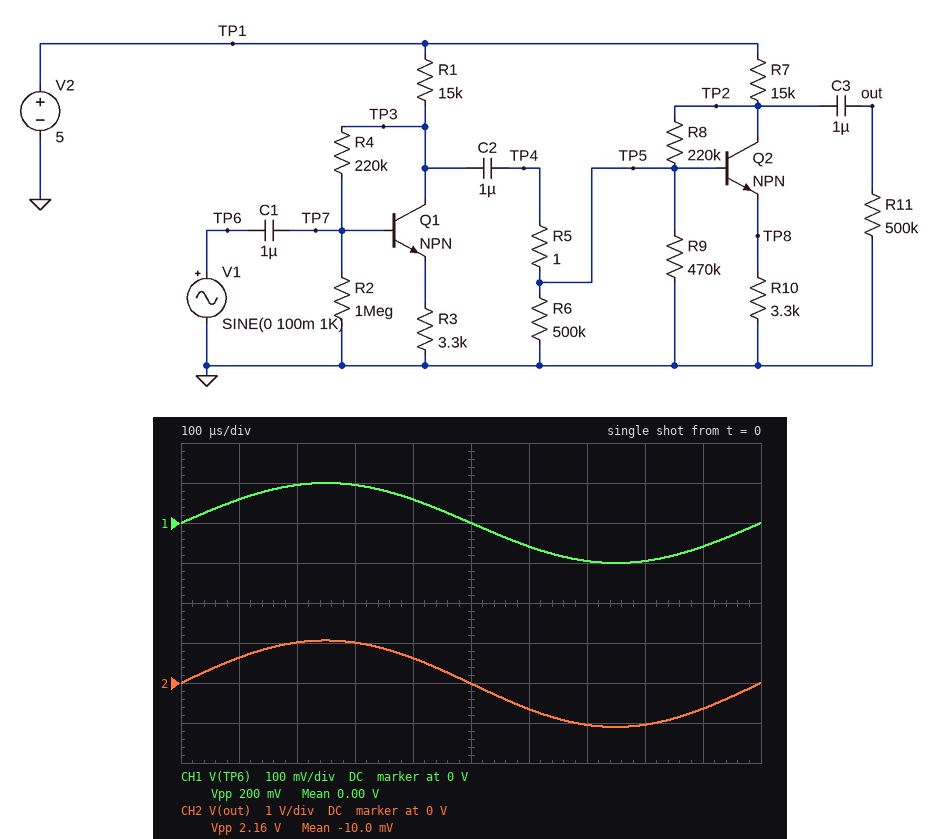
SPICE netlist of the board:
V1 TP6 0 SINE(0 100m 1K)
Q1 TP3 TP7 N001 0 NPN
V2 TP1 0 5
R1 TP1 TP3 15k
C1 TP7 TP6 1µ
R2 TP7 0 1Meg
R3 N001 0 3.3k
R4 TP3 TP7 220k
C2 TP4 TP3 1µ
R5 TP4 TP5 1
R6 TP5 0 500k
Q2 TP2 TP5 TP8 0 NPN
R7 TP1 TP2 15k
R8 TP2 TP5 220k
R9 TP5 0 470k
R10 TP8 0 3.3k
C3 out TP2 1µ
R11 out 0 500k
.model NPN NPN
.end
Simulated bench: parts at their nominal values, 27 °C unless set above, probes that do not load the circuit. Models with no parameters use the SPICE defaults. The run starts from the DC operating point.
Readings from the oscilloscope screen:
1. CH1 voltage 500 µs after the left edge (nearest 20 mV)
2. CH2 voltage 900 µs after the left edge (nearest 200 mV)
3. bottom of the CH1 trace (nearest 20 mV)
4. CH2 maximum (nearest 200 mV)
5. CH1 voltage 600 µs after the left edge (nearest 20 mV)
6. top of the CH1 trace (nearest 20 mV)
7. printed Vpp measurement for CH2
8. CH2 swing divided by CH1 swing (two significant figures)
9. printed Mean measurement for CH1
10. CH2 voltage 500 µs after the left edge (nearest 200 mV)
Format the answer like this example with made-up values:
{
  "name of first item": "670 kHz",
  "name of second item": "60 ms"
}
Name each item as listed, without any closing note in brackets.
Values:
{
  "CH1 voltage 500 µs after the left edge": "0 V",
  "CH2 voltage 900 µs after the left edge": "-600 mV",
  "bottom of the CH1 trace": "-100 mV",
  "CH2 maximum": "1.0 V",
  "CH1 voltage 600 µs after the left edge": "-60 mV",
  "top of the CH1 trace": "100 mV",
  "printed Vpp measurement for CH2": "2.16 V",
  "CH2 swing divided by CH1 swing": "11",
  "printed Mean measurement for CH1": "0.00 V",
  "CH2 voltage 500 µs after the left edge": "0 V"
}
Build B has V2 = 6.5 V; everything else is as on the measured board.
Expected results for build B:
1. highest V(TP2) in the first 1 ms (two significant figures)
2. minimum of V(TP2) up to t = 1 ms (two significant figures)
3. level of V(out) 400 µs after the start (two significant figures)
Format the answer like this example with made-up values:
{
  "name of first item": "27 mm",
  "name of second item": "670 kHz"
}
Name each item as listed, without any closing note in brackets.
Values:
{
  "highest V(TP2) in the first 1 ms": "4.3 V",
  "minimum of V(TP2) up to t = 1 ms": "2.1 V",
  "level of V(out) 400 µs after the start": "640 mV"
}
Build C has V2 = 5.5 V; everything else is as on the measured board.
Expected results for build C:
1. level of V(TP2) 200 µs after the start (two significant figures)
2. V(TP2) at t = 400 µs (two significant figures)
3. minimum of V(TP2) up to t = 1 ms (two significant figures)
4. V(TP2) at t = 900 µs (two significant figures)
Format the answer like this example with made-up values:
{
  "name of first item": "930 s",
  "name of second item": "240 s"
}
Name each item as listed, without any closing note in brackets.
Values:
{
  "level of V(TP2) 200 µs after the start": "3.9 V",
  "V(TP2) at t = 400 µs": "3.5 V",
  "minimum of V(TP2) up to t = 1 ms": "1.7 V",
  "V(TP2) at t = 900 µs": "2.2 V"
}
